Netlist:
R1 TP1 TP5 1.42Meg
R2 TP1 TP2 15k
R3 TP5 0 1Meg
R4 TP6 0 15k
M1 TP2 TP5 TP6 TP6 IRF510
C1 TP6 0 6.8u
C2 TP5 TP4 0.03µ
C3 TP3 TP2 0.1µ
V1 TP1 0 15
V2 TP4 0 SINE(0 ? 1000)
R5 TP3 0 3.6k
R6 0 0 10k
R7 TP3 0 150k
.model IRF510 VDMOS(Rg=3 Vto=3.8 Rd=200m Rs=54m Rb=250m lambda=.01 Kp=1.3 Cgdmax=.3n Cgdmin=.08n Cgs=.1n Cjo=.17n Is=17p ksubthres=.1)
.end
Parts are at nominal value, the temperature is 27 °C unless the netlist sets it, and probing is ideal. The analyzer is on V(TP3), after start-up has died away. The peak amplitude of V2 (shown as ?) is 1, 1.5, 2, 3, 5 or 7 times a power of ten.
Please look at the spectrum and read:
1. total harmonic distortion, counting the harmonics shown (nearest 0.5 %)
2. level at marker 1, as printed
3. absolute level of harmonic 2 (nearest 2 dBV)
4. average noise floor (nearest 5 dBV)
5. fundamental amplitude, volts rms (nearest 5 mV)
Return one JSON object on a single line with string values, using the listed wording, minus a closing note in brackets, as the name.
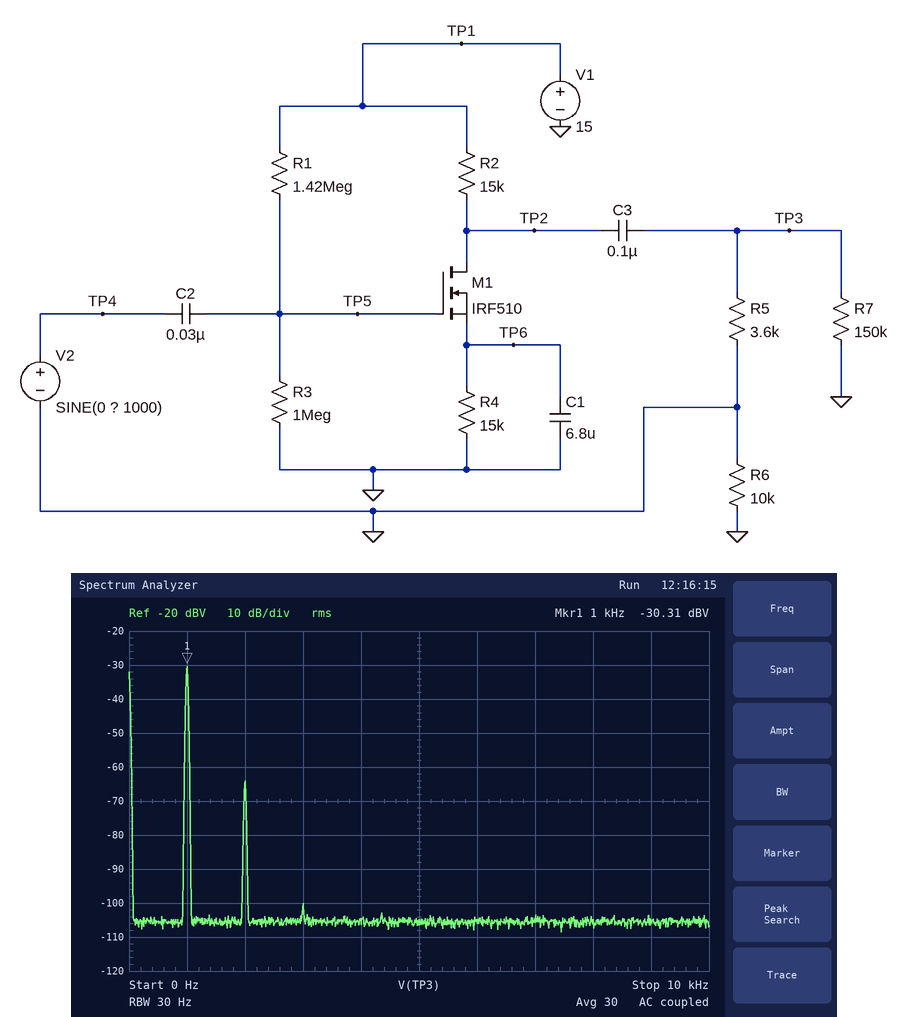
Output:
{"total harmonic distortion, counting the harmonics shown": "2.0 %", "level at marker 1, as printed": "-30.31 dBV", "absolute level of harmonic 2": "-64 dBV", "average noise floor": "-105 dBV", "fundamental amplitude, volts rms": "30 mV"}
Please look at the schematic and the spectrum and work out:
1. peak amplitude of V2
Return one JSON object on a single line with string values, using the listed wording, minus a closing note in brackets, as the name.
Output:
{"peak amplitude of V2": "5 mV"}
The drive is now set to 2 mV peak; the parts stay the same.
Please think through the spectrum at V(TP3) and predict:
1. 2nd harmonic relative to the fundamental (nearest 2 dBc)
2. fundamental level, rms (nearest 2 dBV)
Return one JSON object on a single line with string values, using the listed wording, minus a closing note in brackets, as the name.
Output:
{"2nd harmonic relative to the fundamental": "-42 dBc", "fundamental level, rms": "-38 dBV"}
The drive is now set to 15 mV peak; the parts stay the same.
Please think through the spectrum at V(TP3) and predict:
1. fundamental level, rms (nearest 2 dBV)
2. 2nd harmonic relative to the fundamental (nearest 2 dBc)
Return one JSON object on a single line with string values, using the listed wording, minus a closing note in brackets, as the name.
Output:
{"fundamental level, rms": "-20 dBV", "2nd harmonic relative to the fundamental": "-24 dBc"}
